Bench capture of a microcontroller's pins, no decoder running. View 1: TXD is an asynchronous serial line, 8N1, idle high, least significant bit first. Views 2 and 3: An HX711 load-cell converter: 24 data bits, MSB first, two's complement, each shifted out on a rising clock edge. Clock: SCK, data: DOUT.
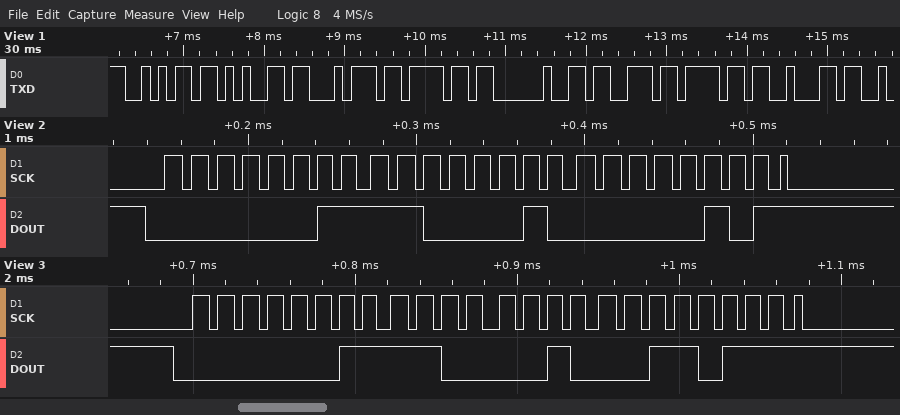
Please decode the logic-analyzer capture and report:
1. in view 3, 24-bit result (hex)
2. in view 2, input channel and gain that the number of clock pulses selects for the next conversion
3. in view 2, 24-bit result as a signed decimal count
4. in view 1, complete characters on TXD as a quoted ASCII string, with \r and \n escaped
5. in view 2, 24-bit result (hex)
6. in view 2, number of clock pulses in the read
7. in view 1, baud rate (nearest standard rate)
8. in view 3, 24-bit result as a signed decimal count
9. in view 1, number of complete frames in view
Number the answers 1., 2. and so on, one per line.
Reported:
1. 0x03C237
2. channel A, gain 128
3. 246277
4. "jeto sob"
5. 0x03C205
6. 25
7. 9600 baud
8. 246327
9. 8
